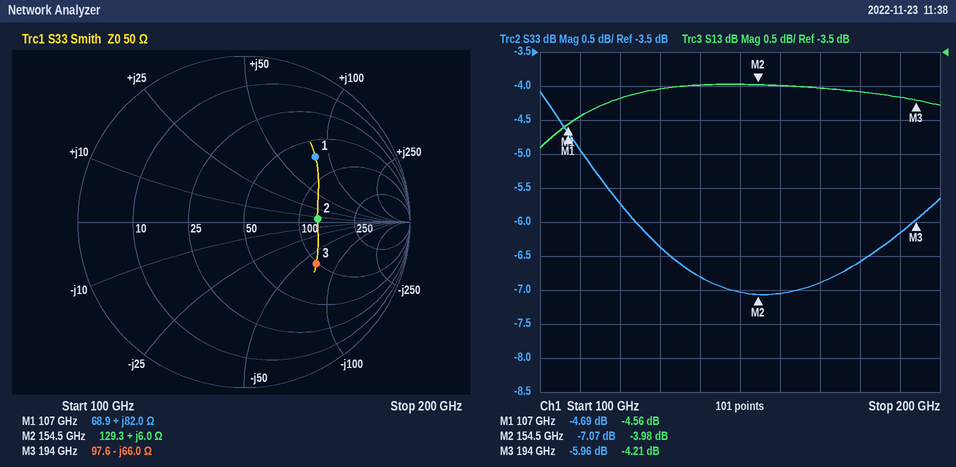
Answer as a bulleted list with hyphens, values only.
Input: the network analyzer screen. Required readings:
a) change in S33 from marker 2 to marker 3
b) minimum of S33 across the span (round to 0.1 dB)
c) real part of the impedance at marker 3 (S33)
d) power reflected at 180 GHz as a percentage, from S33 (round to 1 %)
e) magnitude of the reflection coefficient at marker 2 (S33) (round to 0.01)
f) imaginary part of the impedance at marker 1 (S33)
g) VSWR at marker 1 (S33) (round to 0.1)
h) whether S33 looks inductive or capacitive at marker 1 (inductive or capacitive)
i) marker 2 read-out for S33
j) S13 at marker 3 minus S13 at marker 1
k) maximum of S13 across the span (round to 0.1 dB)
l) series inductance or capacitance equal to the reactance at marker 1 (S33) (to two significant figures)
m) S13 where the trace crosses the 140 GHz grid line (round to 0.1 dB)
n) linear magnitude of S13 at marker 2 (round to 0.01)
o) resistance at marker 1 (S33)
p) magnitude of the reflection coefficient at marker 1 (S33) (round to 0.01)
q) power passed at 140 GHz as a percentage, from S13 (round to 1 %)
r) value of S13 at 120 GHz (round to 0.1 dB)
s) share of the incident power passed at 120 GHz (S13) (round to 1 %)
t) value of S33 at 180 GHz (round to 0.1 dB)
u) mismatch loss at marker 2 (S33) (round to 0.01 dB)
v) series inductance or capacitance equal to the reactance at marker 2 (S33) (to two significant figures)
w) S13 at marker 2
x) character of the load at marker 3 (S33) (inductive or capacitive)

- 1.11 dB
- -7.1 dB
- 97.6 Ω
- 22 %
- 0.44
- +82.0 Ω
- 3.8
- inductive
- -7.07 dB
- 0.35 dB
- -4.0 dB
- 120 pH
- -4.0 dB
- 0.63
- 68.9 Ω
- 0.58
- 40 %
- -4.2 dB
- 38 %
- -6.6 dB
- 0.95 dB
- 6.2 pH
- -3.98 dB
- capacitive
